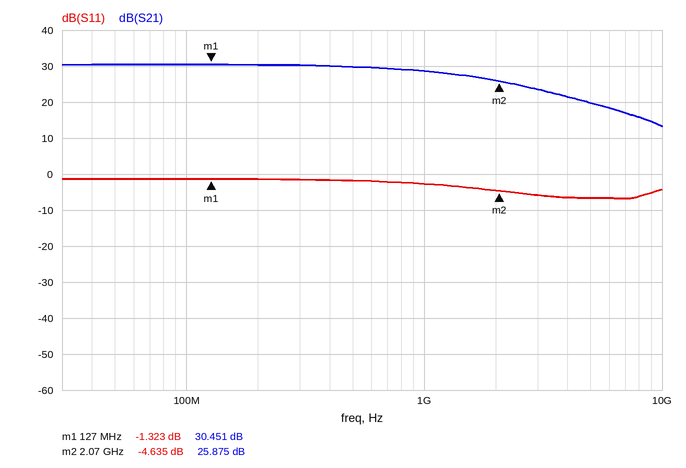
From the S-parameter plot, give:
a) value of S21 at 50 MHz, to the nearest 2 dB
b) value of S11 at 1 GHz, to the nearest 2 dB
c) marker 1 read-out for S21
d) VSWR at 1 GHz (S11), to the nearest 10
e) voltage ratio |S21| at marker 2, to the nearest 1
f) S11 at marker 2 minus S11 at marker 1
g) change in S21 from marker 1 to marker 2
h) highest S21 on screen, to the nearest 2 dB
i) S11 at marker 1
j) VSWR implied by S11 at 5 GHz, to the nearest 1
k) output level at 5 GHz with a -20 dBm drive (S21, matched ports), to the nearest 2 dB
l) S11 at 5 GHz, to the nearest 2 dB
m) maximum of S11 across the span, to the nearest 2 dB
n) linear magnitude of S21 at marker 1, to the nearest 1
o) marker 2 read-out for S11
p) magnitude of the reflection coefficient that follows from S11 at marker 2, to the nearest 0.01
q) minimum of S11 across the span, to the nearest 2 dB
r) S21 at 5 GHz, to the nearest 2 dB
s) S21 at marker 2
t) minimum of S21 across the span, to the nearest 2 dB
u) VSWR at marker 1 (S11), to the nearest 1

30 dB
-2 dB
30.451 dB
10
20
-3.312 dB
-4.576 dB
30 dB
-1.323 dB
3
0 dBm
-6 dB
-2 dB
33
-4.635 dB
0.59
-6 dB
20 dB
25.875 dB
14 dB
13
